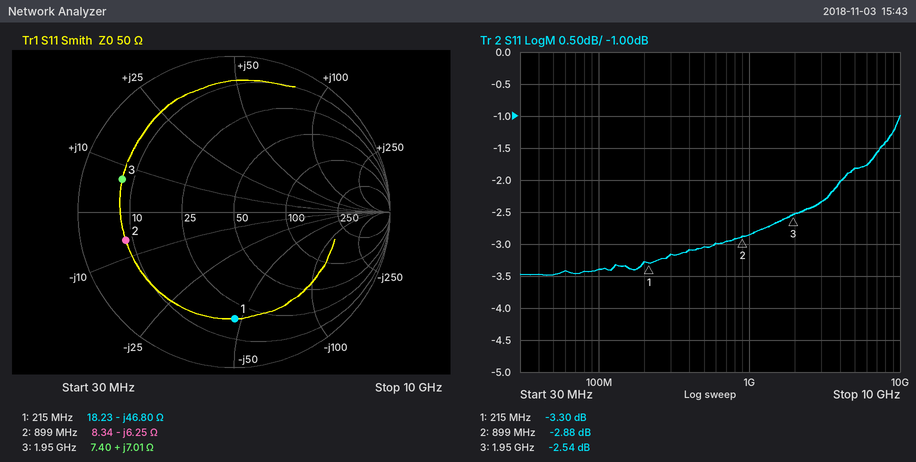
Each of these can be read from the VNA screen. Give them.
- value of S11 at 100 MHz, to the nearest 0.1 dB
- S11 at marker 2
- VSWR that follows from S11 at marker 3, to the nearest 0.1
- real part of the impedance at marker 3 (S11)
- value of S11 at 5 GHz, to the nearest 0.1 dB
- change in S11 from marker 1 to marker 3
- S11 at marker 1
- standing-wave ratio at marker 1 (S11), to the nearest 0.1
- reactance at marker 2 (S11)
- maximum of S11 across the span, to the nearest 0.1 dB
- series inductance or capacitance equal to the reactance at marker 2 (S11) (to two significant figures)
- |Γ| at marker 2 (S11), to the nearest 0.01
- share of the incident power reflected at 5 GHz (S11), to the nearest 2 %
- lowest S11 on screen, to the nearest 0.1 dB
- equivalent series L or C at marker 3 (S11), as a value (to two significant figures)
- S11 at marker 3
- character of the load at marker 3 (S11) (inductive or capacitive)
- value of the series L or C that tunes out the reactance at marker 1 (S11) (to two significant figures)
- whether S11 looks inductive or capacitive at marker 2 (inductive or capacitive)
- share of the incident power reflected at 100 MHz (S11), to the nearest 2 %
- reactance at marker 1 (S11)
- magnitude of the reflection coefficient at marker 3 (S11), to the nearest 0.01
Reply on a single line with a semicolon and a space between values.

-3.4 dB; -2.88 dB; 6.9; 7.40 Ω; -1.8 dB; 0.76 dB; -3.30 dB; 5.3; -6.25 Ω; -1.0 dB; 28 pF; 0.72; 66 %; -3.5 dB; 570 pH; -2.54 dB; inductive; 35 nH; capacitive; 46 %; -46.80 Ω; 0.75
